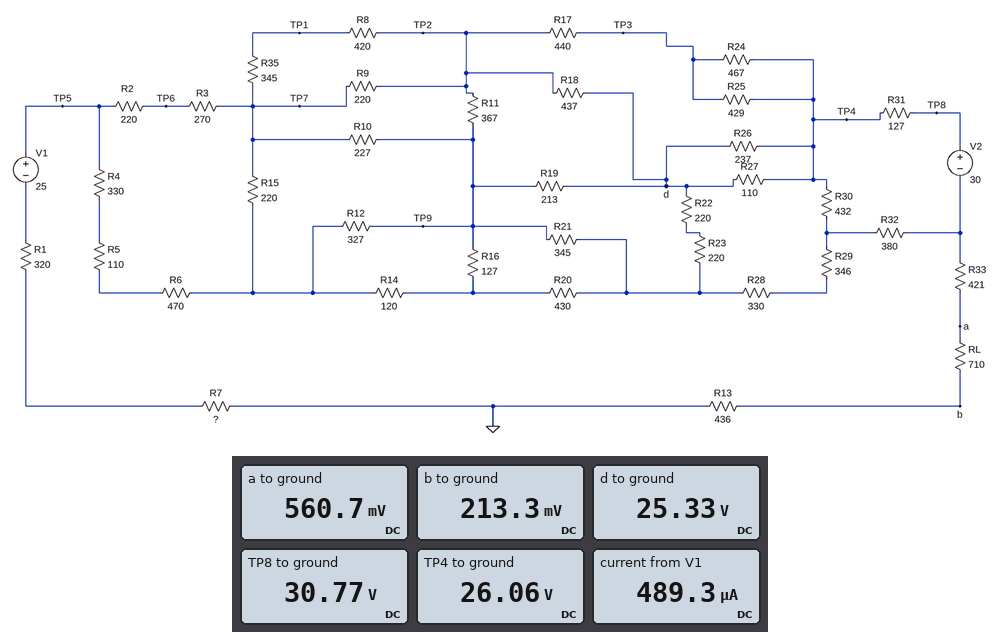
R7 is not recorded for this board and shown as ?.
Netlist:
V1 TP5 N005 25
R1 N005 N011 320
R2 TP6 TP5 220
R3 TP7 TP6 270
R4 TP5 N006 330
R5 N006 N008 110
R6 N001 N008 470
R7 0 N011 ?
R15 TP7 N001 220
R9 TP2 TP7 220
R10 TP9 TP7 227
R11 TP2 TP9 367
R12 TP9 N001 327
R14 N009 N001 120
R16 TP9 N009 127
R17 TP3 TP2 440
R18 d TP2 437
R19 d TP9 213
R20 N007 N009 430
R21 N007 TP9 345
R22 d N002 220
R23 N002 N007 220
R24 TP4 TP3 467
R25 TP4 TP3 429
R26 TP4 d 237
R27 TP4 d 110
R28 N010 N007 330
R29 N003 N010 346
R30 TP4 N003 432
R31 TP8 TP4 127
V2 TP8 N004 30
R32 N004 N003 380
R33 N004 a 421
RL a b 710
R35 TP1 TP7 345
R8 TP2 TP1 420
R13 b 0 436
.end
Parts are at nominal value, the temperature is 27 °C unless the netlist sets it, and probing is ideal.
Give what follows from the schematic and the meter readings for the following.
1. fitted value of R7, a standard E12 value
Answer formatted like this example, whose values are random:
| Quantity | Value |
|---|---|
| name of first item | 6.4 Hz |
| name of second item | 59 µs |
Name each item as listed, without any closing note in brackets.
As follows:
| Quantity | Value |
|---|---|
| fitted value of R7, a standard E12 value | 150 Ω |
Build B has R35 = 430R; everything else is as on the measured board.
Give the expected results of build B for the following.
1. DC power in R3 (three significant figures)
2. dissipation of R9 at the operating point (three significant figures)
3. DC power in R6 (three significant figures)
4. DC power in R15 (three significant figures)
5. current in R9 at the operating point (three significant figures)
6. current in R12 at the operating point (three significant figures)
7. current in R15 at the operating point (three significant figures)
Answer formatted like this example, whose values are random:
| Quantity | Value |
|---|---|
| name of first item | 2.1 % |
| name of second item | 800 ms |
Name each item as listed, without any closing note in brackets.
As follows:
| Quantity | Value |
|---|---|
| DC power in R3 | 8.41 µW |
| dissipation of R9 at the operating point | 294 µW |
| DC power in R6 | 46.2 µW |
| DC power in R15 | 180 µW |
| current in R9 at the operating point | 1.16 mA |
| current in R12 at the operating point | 102 µA |
| current in R15 at the operating point | 904 µA |
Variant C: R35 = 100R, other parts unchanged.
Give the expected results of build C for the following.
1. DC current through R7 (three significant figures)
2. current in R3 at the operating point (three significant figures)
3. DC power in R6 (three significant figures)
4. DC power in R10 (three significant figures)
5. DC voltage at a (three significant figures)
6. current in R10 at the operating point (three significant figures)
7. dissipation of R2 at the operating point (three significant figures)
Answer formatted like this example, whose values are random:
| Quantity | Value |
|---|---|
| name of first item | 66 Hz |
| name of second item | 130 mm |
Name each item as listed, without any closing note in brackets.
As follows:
| Quantity | Value |
|---|---|
| DC current through R7 | 486 µA |
| current in R3 at the operating point | 170 µA |
| DC power in R6 | 46.8 µW |
| DC power in R10 | 132 µW |
| DC voltage at a | 557 mV |
| current in R10 at the operating point | 763 µA |
| dissipation of R2 at the operating point | 6.39 µW |
